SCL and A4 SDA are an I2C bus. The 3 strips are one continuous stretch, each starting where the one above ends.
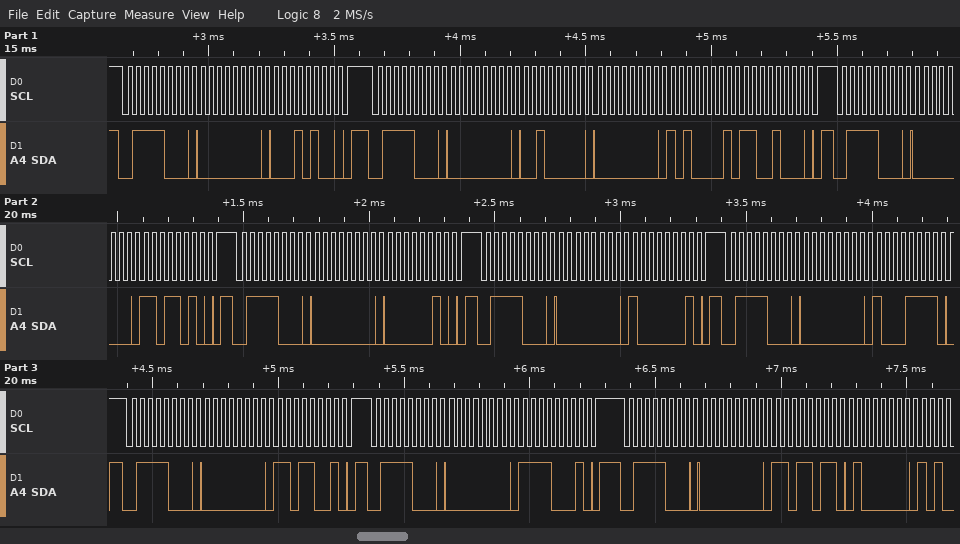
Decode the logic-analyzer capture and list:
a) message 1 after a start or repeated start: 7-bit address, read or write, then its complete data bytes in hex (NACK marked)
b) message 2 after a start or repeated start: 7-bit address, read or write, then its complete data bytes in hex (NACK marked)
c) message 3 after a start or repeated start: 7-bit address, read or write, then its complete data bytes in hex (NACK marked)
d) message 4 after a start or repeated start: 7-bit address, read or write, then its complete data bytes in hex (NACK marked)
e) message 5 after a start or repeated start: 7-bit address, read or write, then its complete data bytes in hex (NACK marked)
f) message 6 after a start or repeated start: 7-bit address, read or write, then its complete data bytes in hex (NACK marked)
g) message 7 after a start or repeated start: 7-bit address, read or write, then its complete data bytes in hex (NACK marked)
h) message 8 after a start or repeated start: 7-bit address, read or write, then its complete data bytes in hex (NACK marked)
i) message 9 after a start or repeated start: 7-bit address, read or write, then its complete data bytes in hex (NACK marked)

0x3C write: 00 14
0x3C write: 00 20 00 A1 C8
0x3C write: 00 DA
0x3C write: 00 02
0x3C write: 00 81
0x3C write: 00 8F
0x3C write: 00 D9
0x3C write: 00 F1
0x3C write: 00 DB 40
